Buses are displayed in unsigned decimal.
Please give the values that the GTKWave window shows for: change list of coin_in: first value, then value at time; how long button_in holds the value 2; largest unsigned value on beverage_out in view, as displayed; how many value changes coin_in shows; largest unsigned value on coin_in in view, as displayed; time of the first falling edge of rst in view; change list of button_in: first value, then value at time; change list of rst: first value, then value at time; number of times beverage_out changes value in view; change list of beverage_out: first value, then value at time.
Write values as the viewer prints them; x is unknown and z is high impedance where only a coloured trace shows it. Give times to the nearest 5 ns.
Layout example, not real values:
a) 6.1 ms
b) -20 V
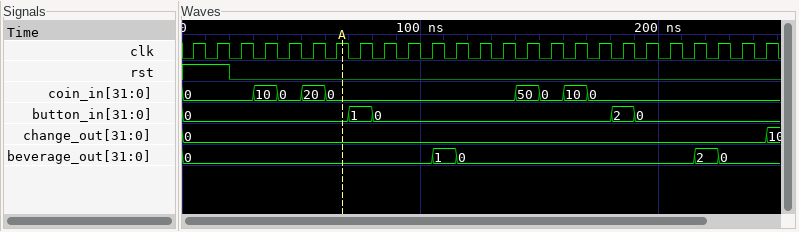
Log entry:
a) 0, 10 at 30 ns, 0 at 40 ns, 20 at 50 ns, 0 at 60 ns, 50 at 140 ns, 0 at 150 ns, 10 at 160 ns, 0 at 170 ns
b) 10 ns
c) 2
d) 8
e) 50
f) 20 ns
g) 0, 1 at 70 ns, 0 at 80 ns, 2 at 180 ns, 0 at 190 ns
h) 1, 0 at 20 ns
i) 4
j) 0, 1 at 105 ns, 0 at 115 ns, 2 at 215 ns, 0 at 225 ns
